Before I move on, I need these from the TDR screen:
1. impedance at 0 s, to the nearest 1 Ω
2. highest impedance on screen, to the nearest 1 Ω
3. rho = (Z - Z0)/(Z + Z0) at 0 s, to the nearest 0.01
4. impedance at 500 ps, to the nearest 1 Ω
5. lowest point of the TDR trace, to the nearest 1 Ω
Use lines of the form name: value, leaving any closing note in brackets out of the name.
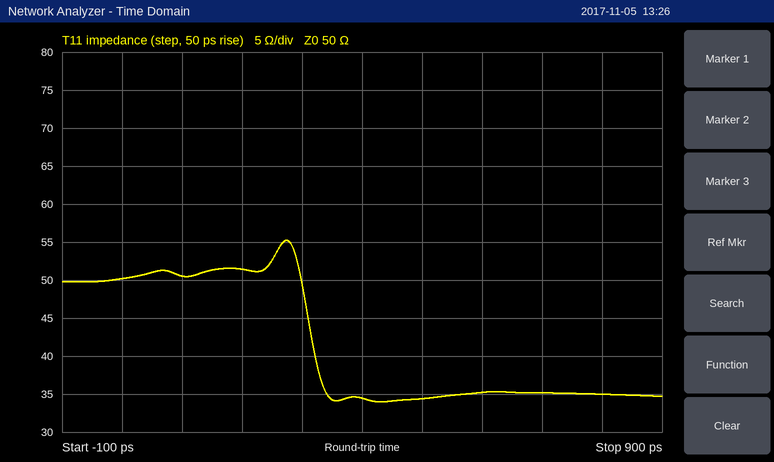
impedance at 0 s, to the nearest 1 Ω: 50 Ω
highest impedance on screen, to the nearest 1 Ω: 55 Ω
rho = (Z - Z0)/(Z + Z0) at 0 s, to the nearest 0.01: 0.00
impedance at 500 ps, to the nearest 1 Ω: 34 Ω
lowest point of the TDR trace, to the nearest 1 Ω: 34 Ω
